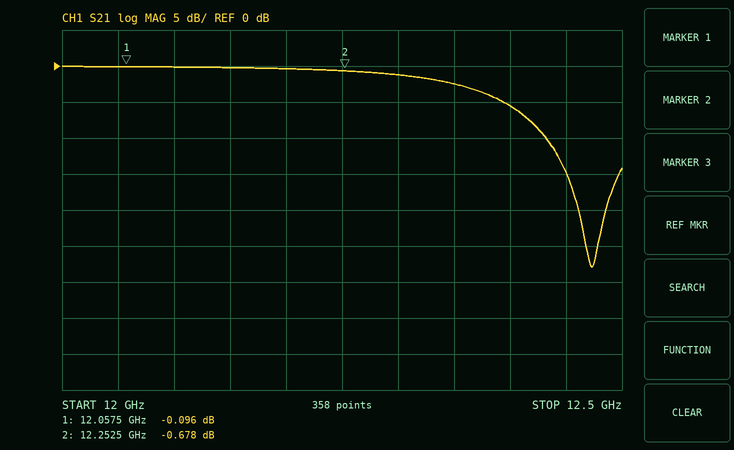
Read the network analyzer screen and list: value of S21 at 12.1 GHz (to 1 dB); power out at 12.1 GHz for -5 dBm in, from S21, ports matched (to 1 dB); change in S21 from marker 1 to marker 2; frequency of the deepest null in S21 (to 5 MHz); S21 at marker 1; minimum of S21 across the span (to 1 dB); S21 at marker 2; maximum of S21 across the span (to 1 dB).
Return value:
0 dB
-5 dBm
-0.582 dB
12.475 GHz
-0.096 dB
-28 dB
-0.678 dB
0 dB
